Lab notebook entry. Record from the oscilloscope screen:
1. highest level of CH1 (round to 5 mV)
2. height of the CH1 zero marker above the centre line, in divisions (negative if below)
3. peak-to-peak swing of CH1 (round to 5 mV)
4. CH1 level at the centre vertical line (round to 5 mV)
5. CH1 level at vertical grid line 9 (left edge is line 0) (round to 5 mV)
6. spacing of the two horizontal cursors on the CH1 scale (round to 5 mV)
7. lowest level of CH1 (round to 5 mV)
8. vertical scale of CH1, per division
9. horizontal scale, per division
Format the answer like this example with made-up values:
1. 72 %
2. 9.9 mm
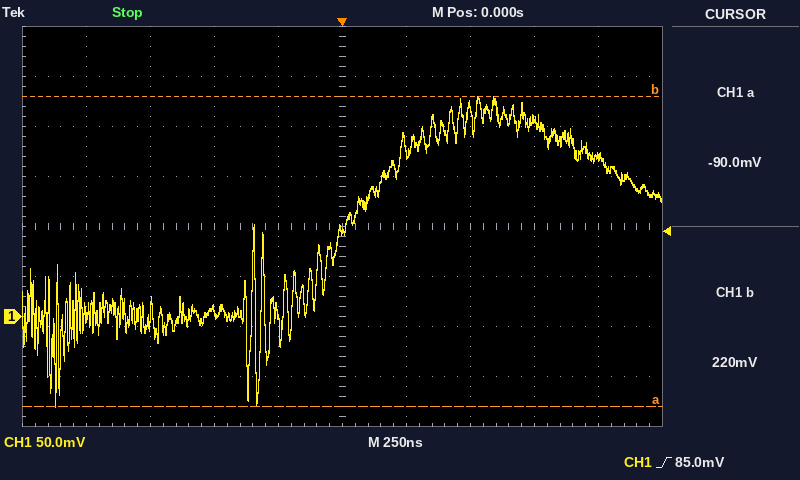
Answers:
1. 220 mV
2. -1.8 div
3. 310 mV
4. 85 mV
5. 160 mV
6. 310 mV
7. -90 mV
8. 50 mV
9. 250 ns
